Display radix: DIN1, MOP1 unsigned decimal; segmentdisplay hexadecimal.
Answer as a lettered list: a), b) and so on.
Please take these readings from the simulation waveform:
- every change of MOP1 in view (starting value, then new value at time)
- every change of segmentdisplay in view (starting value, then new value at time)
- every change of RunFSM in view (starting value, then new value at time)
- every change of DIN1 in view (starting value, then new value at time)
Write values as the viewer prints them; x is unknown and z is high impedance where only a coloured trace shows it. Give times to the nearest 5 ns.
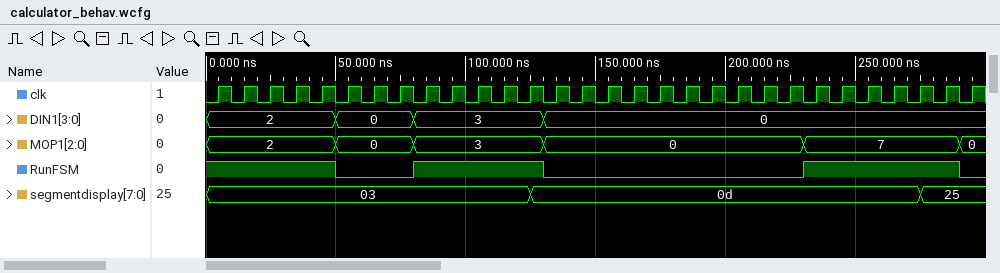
a) 2, 0 at 50 ns, 3 at 80 ns, 0 at 130 ns, 7 at 230 ns, 0 at 290 ns
b) 03, 0d at 125 ns, 25 at 275 ns
c) 1, 0 at 50 ns, 1 at 80 ns, 0 at 130 ns, 1 at 230 ns, 0 at 290 ns
d) 2, 0 at 50 ns, 3 at 80 ns, 0 at 130 ns
